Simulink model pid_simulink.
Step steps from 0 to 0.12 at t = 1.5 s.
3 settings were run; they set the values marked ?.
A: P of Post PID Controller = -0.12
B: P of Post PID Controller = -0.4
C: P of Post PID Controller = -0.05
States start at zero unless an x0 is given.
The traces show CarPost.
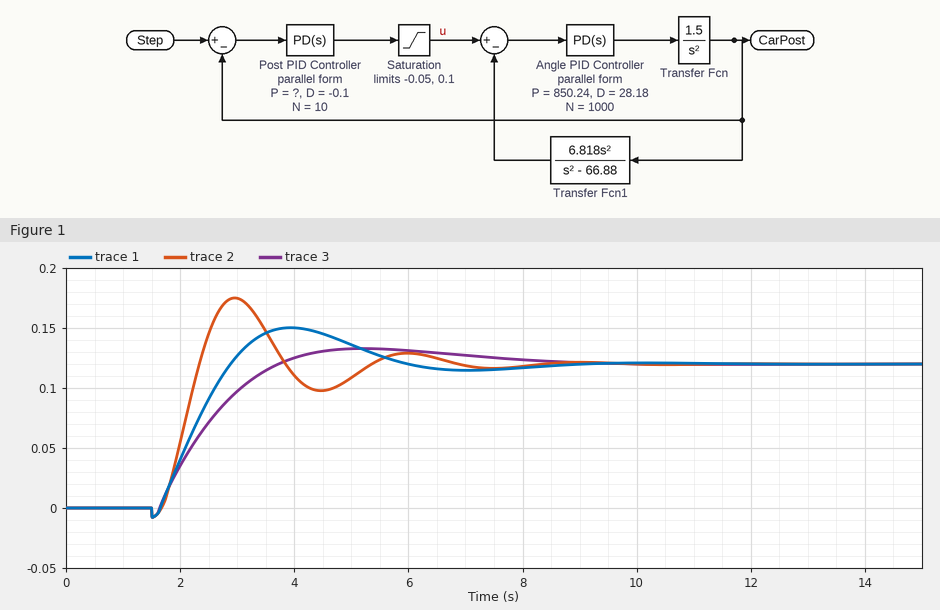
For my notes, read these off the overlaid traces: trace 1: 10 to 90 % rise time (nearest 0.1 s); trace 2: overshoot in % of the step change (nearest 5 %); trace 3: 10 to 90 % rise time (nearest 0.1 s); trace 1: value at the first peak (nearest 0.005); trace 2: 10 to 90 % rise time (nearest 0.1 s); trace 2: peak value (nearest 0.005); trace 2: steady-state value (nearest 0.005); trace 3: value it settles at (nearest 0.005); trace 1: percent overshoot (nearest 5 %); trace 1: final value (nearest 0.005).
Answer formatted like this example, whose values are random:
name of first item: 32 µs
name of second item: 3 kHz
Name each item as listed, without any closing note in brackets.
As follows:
trace 1: 10 to 90 % rise time: 1.0 s
trace 2: overshoot in % of the step change: 45 %
trace 3: 10 to 90 % rise time: 1.5 s
trace 1: value at the first peak: 0.150
trace 2: 10 to 90 % rise time: 0.5 s
trace 2: peak value: 0.175
trace 2: steady-state value: 0.120
trace 3: value it settles at: 0.120
trace 1: percent overshoot: 25 %
trace 1: final value: 0.120
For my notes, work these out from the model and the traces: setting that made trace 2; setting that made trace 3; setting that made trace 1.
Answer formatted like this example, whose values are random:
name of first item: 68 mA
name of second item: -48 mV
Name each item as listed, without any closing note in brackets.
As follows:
setting that made trace 2: B
setting that made trace 3: C
setting that made trace 1: A
